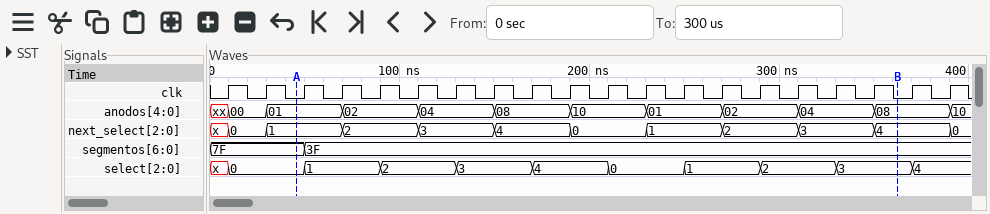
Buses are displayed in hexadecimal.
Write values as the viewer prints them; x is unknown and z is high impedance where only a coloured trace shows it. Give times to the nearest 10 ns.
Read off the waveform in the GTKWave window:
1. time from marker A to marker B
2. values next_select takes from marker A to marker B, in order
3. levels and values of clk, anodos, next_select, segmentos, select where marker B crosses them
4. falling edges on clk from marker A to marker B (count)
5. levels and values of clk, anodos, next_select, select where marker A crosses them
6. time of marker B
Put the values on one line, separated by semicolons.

320 ns; 1, 2, 3, 4, 0, 1, 2, 3, 4; clk=0, anodos=08, next_select=4, segmentos=3F, select=3; 16; clk=0, anodos=01, next_select=1, select=0; 360 ns
